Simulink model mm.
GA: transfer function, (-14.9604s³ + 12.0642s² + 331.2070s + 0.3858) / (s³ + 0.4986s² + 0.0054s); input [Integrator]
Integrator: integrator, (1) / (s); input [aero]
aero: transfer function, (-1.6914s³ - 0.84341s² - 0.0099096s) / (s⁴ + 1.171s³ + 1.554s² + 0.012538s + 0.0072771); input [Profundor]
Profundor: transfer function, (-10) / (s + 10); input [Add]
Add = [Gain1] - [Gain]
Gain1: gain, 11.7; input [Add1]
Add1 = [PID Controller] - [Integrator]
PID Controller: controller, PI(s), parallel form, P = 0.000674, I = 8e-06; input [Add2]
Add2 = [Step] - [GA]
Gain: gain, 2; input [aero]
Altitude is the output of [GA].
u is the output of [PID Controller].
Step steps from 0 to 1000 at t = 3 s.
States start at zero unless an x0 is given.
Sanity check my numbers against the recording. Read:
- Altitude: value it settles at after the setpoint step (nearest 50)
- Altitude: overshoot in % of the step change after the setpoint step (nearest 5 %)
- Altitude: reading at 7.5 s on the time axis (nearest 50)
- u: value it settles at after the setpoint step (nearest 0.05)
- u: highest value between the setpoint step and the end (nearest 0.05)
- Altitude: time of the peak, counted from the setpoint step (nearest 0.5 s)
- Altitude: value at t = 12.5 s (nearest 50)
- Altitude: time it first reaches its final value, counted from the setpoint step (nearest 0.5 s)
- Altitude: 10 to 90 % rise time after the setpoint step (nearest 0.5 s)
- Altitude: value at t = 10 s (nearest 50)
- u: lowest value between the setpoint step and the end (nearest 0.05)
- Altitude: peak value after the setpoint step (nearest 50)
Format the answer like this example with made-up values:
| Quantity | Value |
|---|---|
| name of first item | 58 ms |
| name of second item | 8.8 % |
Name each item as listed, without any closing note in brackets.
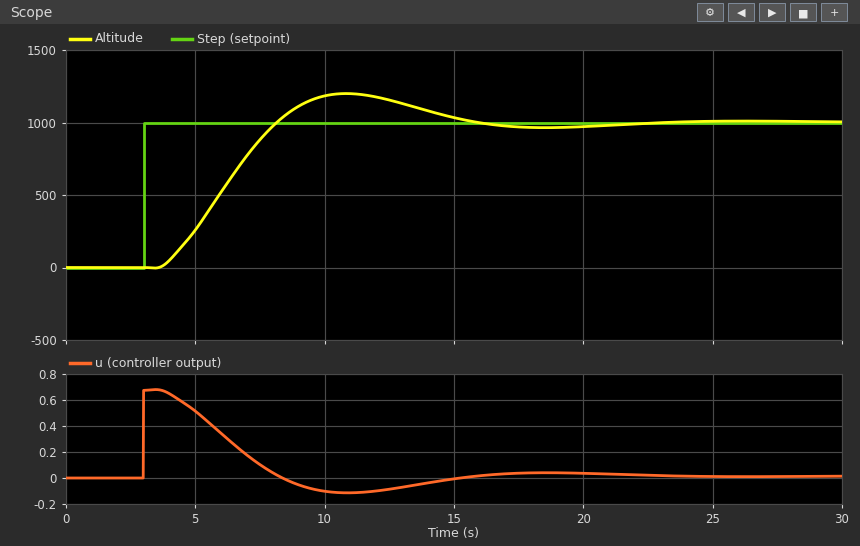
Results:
| Quantity | Value |
|---|---|
| Altitude: value it settles at after the setpoint step | 1000 |
| Altitude: overshoot in % of the step change after the setpoint step | 20 % |
| Altitude: reading at 7.5 s on the time axis | 900 |
| u: value it settles at after the setpoint step | 0.00 |
| u: highest value between the setpoint step and the end | 0.70 |
| Altitude: time of the peak, counted from the setpoint step | 8.0 s |
| Altitude: value at t = 12.5 s | 1150 |
| Altitude: time it first reaches its final value, counted from the setpoint step | 5.0 s |
| Altitude: 10 to 90 % rise time after the setpoint step | 3.5 s |
| Altitude: value at t = 10 s | 1200 |
| u: lowest value between the setpoint step and the end | -0.10 |
| Altitude: peak value after the setpoint step | 1200 |
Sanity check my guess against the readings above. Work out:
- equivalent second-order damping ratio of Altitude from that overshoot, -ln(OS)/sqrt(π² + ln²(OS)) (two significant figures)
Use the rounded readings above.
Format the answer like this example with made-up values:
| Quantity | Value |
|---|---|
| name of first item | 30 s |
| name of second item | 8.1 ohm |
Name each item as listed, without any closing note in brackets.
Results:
| Quantity | Value |
|---|---|
| equivalent second-order damping ratio of Altitude from that overshoot, -ln(OS)/sqrt(π² + ln²(OS)) | 0.46 |
